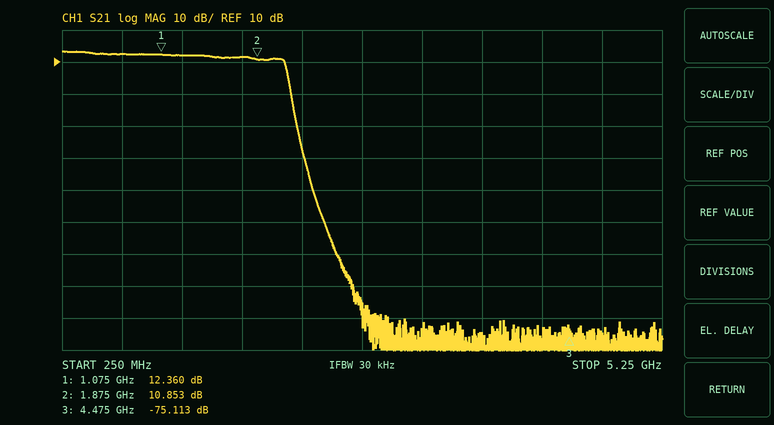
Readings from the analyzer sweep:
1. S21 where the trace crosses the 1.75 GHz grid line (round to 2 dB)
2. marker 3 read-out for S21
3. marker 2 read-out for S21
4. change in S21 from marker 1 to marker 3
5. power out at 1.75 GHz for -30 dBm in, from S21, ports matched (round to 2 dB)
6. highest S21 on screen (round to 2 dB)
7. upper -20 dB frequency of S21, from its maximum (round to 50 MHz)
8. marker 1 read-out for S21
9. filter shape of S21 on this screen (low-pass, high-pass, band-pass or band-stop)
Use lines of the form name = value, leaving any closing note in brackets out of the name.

S21 where the trace crosses the 1.75 GHz grid line = 12 dB
marker 3 read-out for S21 = -75.113 dB
marker 2 read-out for S21 = 10.853 dB
change in S21 from marker 1 to marker 3 = -87.473 dB
power out at 1.75 GHz for -30 dBm in, from S21, ports matched = -18 dBm
highest S21 on screen = 14 dB
upper -20 dB frequency of S21, from its maximum = 2.20 GHz
marker 1 read-out for S21 = 12.360 dB
filter shape of S21 on this screen = low-pass
